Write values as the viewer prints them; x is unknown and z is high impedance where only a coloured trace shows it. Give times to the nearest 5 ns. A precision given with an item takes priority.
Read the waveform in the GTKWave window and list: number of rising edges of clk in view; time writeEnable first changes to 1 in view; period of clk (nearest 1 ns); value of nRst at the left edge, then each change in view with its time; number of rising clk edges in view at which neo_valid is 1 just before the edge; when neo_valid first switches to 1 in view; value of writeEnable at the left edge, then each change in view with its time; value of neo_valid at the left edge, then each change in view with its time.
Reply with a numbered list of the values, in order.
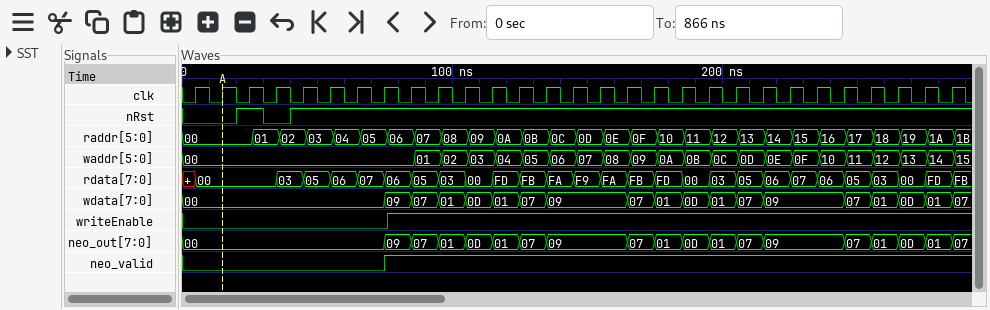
1. 29
2. 75 ns
3. 10 ns
4. 0, 1 at 20 ns, 0 at 30 ns, 1 at 40 ns
5. 21
6. 75 ns
7. 0, 1 at 75 ns
8. 0, 1 at 75 ns
